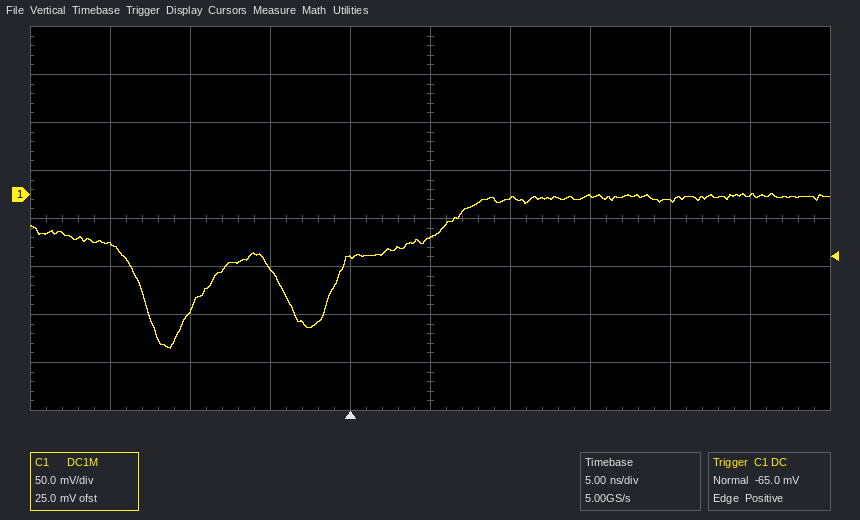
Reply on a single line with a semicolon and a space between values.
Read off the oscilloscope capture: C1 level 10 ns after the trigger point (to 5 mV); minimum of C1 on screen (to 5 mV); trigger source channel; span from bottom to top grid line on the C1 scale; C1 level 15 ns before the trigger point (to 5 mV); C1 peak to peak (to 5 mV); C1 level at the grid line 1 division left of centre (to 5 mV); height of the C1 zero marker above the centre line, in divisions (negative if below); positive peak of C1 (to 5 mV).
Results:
-5 mV; -160 mV; C1; 400 mV; -50 mV; 160 mV; -65 mV; +0.5 div; 0 mV
